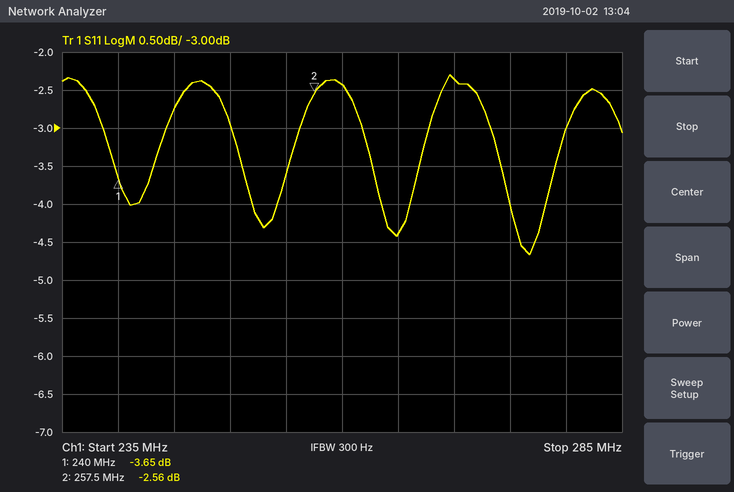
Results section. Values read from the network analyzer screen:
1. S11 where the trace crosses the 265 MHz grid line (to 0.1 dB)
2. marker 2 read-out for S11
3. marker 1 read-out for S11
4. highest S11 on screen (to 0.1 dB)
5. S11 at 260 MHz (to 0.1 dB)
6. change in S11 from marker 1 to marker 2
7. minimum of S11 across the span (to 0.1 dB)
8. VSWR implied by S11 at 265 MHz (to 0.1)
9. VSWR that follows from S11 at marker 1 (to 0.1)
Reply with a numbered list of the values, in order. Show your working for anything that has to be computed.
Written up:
1. -4.4 dB
2. -2.56 dB
3. -3.65 dB
4. -2.3 dB
5. -2.4 dB
6. -2.56 − (-3.65) = 1.09 dB
7. -4.7 dB
8. |Γ| = 10^(-4.4/20) = 0.6026; VSWR = (1 + 0.6026)/(1 − 0.6026) ≈ 4.0
9. (1 + 0.6569)/(1 − 0.6569) ≈ 4.8
